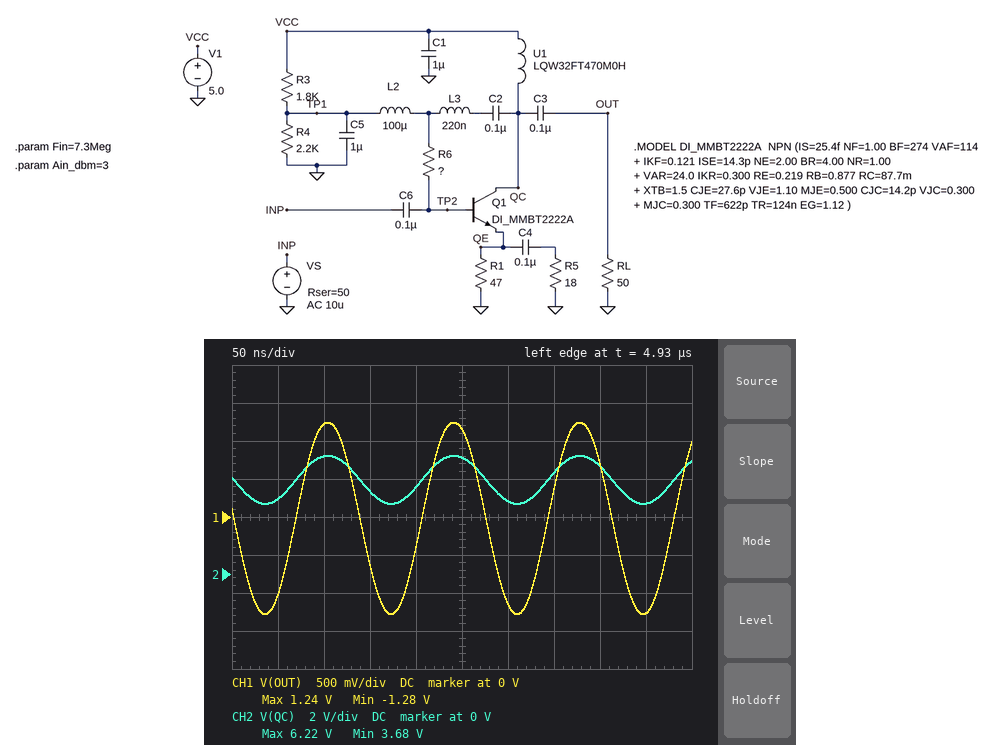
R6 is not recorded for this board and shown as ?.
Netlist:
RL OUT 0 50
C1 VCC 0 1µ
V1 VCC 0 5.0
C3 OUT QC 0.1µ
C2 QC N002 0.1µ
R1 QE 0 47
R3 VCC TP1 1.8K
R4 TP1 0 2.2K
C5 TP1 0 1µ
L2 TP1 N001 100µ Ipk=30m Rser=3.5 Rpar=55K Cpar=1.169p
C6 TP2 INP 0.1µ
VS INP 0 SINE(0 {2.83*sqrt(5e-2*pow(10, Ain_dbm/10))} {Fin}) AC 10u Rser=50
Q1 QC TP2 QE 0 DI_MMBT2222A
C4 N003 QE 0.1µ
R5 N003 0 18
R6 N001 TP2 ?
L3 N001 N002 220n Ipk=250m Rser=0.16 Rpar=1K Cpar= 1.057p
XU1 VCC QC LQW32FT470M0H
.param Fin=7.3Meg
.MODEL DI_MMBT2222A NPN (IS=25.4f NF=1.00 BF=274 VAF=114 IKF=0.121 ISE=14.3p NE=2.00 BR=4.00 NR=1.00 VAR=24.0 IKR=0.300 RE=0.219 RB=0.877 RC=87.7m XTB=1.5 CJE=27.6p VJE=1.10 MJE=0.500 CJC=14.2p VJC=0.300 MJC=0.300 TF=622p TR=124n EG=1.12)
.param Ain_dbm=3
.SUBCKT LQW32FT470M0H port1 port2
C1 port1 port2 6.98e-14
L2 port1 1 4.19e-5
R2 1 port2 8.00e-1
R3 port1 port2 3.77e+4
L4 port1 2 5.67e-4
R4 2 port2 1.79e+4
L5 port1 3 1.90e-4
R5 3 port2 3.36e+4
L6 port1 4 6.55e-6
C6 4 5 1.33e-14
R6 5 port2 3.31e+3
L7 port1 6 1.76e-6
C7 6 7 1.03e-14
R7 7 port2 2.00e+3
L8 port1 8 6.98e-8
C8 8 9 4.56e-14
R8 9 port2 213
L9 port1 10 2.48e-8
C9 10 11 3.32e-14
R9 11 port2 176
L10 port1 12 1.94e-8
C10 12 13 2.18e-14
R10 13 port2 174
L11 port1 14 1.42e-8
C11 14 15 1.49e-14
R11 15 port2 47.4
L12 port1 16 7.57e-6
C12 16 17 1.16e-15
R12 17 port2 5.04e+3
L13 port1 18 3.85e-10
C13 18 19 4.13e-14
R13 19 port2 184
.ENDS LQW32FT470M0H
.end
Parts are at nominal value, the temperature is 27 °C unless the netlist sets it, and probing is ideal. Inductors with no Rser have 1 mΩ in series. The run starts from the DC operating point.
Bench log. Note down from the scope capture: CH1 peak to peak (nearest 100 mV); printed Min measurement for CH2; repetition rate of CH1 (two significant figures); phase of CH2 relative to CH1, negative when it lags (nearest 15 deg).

2.5 V
3.68 V
7.3 MHz
0 deg
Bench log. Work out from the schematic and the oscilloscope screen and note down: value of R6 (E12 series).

220 Ω
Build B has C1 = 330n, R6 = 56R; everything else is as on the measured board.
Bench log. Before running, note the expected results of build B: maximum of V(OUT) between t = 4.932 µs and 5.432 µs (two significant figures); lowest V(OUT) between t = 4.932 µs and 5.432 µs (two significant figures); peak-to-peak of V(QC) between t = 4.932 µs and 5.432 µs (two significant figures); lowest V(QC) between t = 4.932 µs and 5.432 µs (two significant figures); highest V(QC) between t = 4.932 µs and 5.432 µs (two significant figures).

400 mV
-410 mV
810 mV
4.6 V
5.4 V
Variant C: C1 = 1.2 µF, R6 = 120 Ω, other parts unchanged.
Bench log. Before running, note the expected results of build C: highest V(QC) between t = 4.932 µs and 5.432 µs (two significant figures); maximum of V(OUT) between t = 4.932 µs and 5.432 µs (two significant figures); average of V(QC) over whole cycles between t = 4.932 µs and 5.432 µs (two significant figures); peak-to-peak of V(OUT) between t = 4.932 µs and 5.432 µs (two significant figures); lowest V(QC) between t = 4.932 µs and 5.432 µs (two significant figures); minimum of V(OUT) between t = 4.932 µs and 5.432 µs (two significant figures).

5.8 V
820 mV
5.0 V
1.7 V
4.1 V
-840 mV
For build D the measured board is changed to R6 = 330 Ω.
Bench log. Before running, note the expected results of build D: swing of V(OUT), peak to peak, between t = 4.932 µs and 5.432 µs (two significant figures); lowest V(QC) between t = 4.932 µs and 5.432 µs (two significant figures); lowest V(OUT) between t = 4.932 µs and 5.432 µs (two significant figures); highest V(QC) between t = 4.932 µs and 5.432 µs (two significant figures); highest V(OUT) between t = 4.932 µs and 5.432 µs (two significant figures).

3.1 V
3.4 V
-1.6 V
6.5 V
1.5 V
